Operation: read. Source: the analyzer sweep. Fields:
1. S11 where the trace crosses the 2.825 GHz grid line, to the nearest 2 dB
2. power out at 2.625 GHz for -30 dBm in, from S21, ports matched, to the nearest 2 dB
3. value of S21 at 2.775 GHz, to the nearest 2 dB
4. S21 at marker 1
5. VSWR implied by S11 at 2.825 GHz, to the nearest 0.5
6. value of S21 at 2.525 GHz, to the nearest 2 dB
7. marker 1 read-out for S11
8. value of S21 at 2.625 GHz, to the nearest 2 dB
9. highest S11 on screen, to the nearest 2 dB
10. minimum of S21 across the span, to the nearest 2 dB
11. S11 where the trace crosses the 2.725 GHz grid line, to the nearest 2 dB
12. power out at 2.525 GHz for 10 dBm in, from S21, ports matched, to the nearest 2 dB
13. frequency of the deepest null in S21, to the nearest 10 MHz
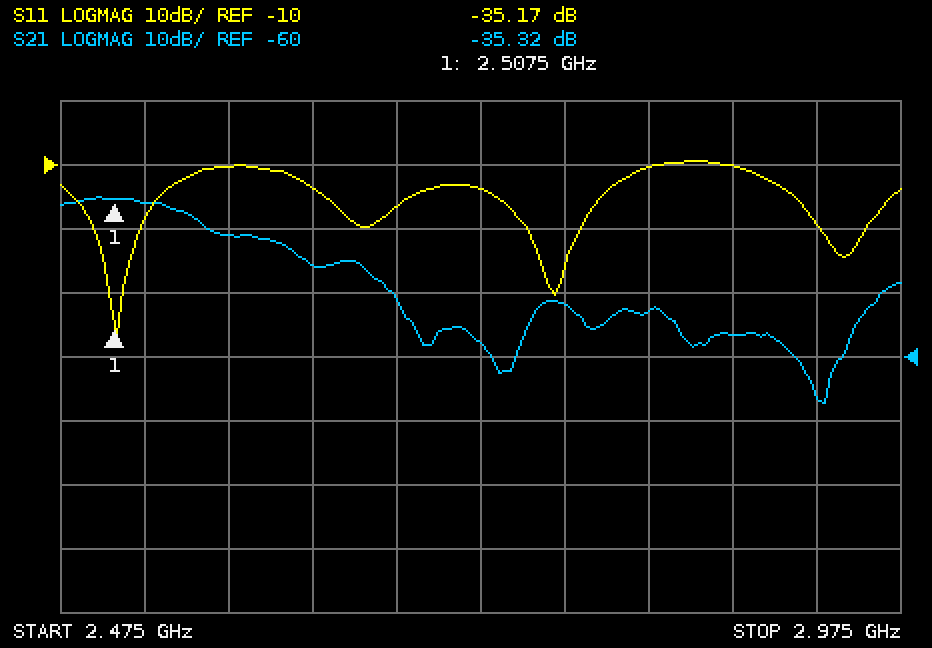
-10 dB
-76 dBm
-52 dB
-35.32 dB
2.0
-36 dB
-35.17 dB
-46 dB
-10 dB
-68 dB
-14 dB
-26 dBm
2.93 GHz
